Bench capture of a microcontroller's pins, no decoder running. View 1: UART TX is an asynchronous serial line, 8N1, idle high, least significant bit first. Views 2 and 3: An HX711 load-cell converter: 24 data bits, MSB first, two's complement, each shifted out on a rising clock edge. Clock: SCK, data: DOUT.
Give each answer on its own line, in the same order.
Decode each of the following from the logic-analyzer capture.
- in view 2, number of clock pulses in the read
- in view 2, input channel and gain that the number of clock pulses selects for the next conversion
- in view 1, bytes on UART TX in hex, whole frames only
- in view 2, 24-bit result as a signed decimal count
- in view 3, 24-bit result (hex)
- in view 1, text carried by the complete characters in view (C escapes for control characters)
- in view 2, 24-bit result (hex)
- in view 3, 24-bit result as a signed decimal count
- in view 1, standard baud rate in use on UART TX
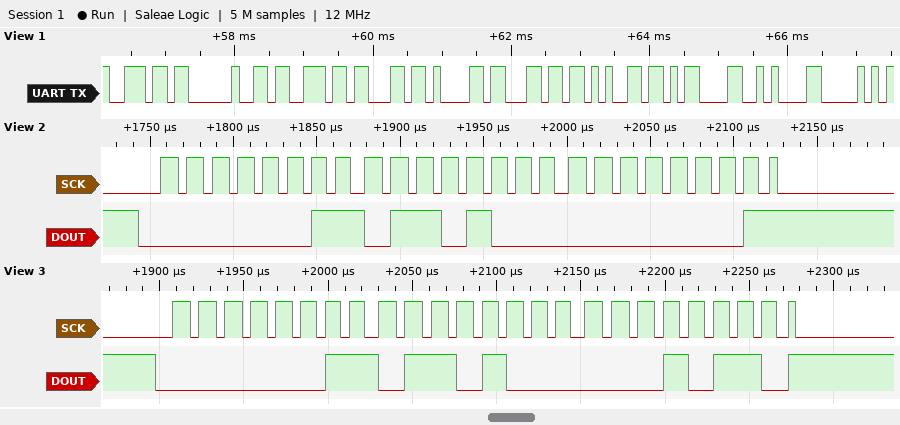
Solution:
25
channel A, gain 128
6E 20 73 63 61 6C 65 0D 0A 50
223233
0x036816
"n scale\r\nP"
0x036801
223254
9600 baud
